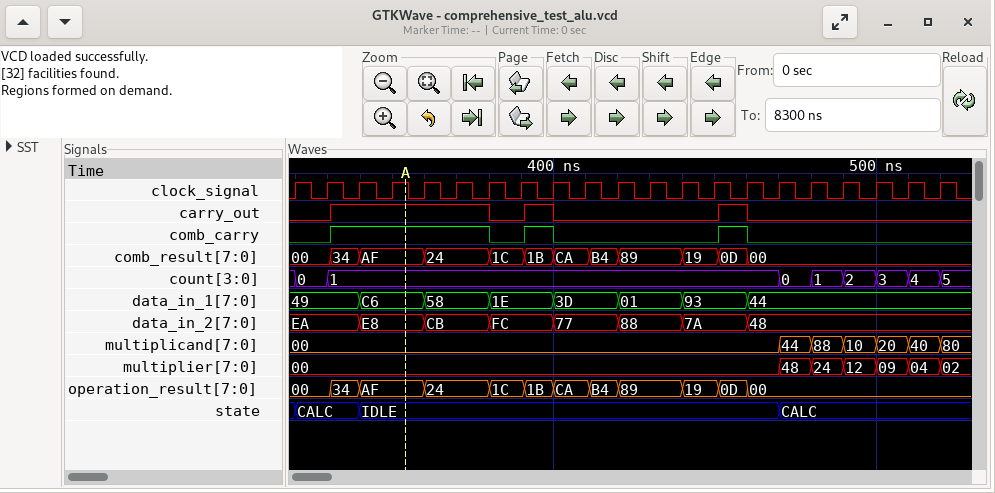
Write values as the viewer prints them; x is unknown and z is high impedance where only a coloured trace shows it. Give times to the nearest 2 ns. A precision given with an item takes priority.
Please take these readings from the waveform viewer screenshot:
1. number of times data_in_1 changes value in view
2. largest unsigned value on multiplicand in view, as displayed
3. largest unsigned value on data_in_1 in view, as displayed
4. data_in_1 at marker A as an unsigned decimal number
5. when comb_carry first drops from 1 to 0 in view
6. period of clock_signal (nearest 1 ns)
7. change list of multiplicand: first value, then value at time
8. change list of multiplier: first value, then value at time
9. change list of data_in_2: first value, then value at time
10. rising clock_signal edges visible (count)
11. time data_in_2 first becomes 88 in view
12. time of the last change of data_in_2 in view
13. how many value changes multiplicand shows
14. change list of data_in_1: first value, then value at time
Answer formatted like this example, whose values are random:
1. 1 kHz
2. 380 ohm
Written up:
1. 7
2. 88
3. C6
4. 198
5. 380 ns
6. 10 ns
7. 00, 44 at 470 ns, 88 at 480 ns, 10 at 490 ns, 20 at 500 ns, 40 at 510 ns, 80 at 520 ns
8. 00, 48 at 470 ns, 24 at 480 ns, 12 at 490 ns, 09 at 500 ns, 04 at 510 ns, 02 at 520 ns
9. EA, E8 at 340 ns, CB at 360 ns, FC at 380 ns, 77 at 400 ns, 88 at 420 ns, 7A at 440 ns, 48 at 460 ns
10. 21
11. 420 ns
12. 460 ns
13. 6
14. 49, C6 at 340 ns, 58 at 360 ns, 1E at 380 ns, 3D at 400 ns, 01 at 420 ns, 93 at 440 ns, 44 at 460 ns
